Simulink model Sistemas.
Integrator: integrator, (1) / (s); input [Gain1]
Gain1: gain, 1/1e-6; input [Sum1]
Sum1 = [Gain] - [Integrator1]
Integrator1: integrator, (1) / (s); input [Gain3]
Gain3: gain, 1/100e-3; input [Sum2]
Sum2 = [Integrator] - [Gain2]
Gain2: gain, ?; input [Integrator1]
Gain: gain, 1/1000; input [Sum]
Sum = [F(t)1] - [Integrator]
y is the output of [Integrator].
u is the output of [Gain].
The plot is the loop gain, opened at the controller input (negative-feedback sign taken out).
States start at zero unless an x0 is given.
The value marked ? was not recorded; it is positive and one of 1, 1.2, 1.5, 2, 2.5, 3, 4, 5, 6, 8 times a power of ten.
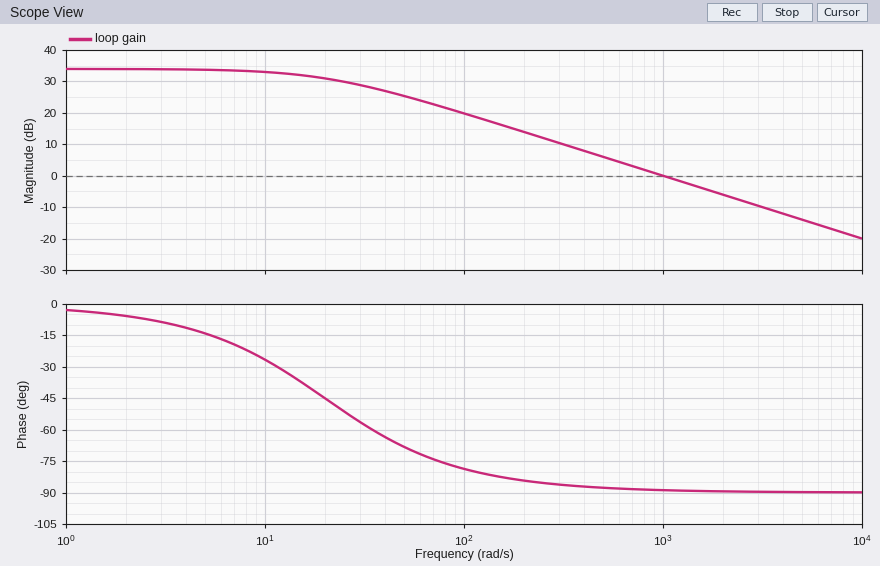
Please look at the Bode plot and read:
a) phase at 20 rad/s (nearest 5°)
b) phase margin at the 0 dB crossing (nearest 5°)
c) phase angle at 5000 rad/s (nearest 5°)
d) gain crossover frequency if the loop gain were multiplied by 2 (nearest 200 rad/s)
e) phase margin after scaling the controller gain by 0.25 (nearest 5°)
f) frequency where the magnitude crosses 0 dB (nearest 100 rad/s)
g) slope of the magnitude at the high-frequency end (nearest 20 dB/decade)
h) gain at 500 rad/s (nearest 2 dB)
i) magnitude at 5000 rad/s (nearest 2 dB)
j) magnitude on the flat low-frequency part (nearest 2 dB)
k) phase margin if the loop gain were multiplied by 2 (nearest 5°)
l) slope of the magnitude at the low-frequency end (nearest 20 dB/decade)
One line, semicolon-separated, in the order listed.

-45°; 90°; -90°; 2000 rad/s; 95°; 1000 rad/s; -20 dB/decade; 6 dB; -14 dB; 34 dB; 90°; 0 dB/decade
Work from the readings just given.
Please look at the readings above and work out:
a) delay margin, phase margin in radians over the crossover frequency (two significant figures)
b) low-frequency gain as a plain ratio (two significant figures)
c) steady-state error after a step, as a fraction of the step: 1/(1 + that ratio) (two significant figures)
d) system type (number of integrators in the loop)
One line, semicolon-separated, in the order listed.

0.0016 s; 50; 0.020; 0
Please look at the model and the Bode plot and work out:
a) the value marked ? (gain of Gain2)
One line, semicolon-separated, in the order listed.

50000
